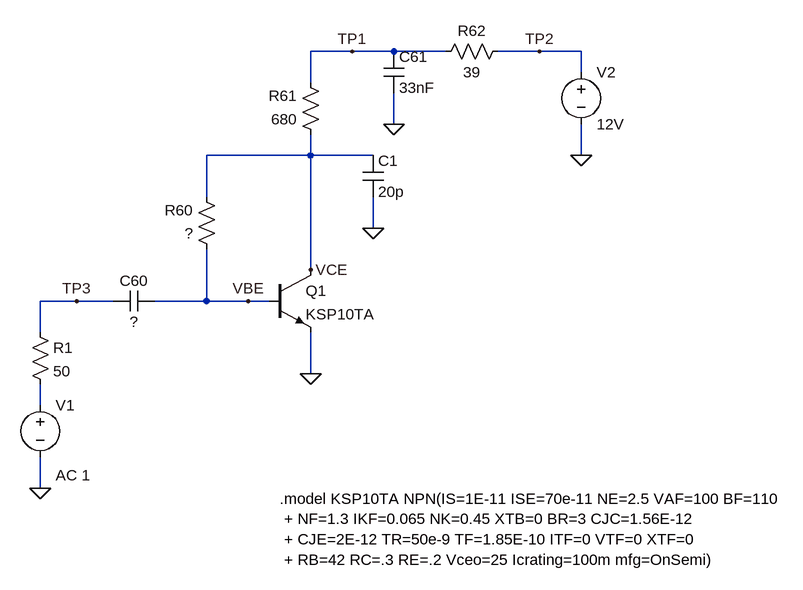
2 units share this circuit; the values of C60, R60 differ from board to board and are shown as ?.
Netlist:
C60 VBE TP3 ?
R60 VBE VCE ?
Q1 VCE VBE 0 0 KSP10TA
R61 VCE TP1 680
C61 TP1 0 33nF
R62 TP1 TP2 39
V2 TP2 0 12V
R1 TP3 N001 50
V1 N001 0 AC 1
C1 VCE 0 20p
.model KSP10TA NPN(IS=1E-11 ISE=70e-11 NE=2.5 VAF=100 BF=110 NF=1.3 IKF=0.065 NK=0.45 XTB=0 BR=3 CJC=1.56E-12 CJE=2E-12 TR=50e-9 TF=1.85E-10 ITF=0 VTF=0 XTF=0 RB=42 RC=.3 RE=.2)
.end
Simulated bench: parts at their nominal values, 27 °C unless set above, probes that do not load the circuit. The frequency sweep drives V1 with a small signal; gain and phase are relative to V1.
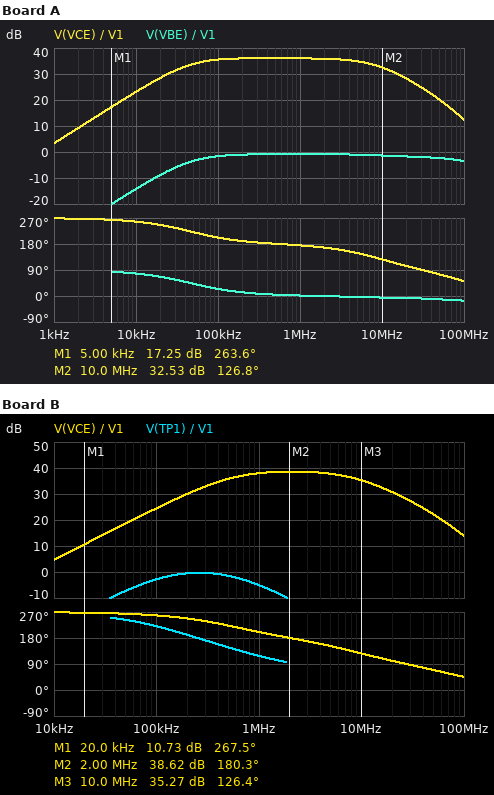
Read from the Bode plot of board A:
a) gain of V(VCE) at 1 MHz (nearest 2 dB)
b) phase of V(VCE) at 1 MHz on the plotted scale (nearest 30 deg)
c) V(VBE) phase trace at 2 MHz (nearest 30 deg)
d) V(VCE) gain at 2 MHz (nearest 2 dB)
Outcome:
36 dB
180 deg
0 deg
36 dB
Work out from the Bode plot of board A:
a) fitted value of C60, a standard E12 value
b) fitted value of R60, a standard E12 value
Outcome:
5.6 nF
150 kΩ
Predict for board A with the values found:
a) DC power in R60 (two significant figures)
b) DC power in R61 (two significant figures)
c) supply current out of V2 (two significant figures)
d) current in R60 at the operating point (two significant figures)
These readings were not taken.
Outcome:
470 µW
11 mW
4.1 mA
56 µA
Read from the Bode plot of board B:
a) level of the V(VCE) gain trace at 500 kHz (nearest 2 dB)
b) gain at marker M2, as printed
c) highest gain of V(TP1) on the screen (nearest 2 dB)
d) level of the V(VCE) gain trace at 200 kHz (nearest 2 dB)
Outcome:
36 dB
38.62 dB
0 dB
30 dB
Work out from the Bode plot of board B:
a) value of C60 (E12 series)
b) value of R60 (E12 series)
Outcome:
1 nF
56 kΩ
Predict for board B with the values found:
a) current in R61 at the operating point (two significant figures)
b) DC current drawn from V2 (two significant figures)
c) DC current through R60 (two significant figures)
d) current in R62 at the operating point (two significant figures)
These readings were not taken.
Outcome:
7.8 mA
7.8 mA
100 µA
7.8 mA
